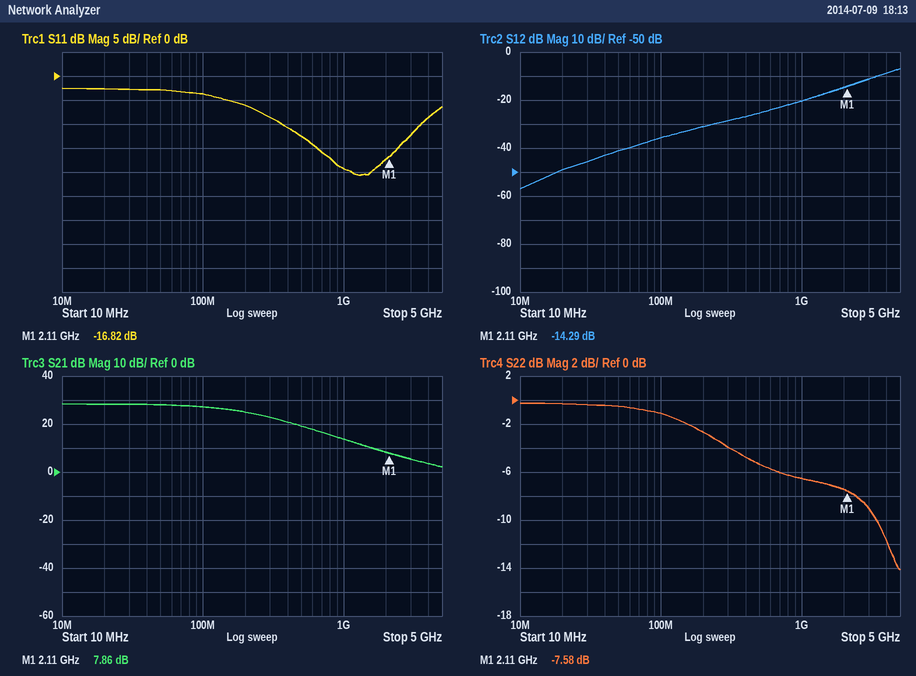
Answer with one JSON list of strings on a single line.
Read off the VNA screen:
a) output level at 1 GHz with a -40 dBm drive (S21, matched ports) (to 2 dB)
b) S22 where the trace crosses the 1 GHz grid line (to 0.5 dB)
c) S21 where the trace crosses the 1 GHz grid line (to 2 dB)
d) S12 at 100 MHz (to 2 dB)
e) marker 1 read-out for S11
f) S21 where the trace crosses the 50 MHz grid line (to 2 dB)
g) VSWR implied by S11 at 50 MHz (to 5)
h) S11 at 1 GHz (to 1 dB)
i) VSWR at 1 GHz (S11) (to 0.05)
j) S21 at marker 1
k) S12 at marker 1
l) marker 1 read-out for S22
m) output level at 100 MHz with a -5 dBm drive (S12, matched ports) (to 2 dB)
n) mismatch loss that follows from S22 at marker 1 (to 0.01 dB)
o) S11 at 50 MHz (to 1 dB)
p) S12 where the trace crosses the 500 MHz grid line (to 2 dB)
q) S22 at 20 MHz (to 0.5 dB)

["-26 dBm", "-6.5 dB", "14 dB", "-36 dB", "-16.82 dB", "28 dB", "5", "-19 dB", "1.25", "7.86 dB", "-14.29 dB", "-7.58 dB", "-40 dBm", "0.83 dB", "-3 dB", "-26 dB", "-0.5 dB"]
